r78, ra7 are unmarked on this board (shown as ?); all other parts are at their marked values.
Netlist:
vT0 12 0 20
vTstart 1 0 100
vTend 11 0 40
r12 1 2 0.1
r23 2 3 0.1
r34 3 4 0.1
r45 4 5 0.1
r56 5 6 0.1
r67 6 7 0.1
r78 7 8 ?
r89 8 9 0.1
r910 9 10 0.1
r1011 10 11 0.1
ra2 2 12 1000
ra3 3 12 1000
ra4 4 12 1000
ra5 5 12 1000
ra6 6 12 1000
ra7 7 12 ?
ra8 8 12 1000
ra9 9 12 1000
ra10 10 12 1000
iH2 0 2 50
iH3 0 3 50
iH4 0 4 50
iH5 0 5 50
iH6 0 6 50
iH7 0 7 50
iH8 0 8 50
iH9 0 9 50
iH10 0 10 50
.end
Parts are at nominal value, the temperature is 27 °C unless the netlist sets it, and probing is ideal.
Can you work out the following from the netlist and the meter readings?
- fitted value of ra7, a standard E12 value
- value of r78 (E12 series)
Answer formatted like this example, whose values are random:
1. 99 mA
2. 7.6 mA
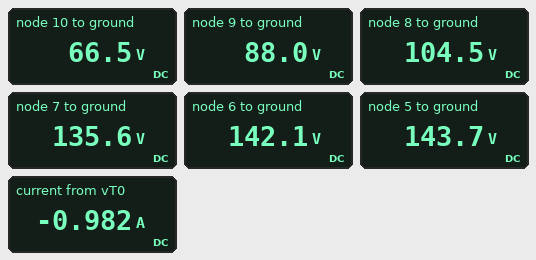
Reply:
1. 560 Ω
2. 0.27 Ω
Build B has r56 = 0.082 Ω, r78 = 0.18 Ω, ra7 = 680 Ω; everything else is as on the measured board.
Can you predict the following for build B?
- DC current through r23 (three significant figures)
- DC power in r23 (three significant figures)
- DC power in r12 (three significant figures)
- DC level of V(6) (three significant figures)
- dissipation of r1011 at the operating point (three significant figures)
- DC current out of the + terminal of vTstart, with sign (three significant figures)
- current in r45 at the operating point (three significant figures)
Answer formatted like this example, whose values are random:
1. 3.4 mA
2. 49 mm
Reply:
1. 124 A
2. 1.54 kW
3. 3.03 kW
4. 138 V
5. 7.56 kW
6. -174 A
7. 24.4 A
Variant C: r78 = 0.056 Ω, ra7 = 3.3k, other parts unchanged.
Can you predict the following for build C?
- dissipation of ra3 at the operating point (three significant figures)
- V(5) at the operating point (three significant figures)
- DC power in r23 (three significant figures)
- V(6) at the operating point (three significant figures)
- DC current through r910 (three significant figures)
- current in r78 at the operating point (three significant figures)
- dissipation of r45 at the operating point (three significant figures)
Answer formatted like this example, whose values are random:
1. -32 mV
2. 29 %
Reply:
1. 11.4 W
2. 133 V
3. 1.18 kW
4. 129 V
5. 241 A
6. 141 A
7. 7.53 W
